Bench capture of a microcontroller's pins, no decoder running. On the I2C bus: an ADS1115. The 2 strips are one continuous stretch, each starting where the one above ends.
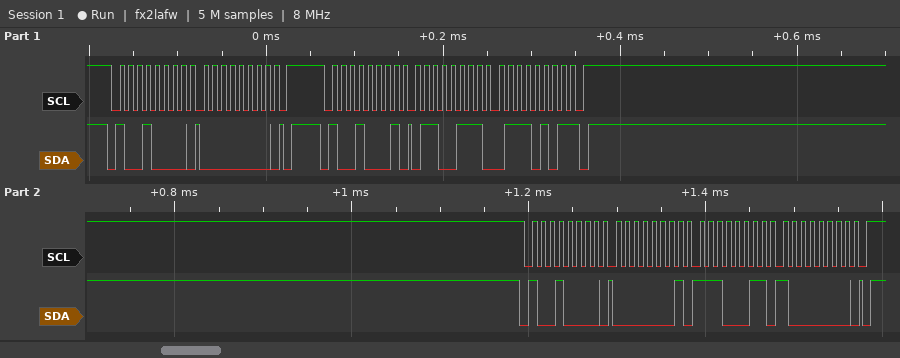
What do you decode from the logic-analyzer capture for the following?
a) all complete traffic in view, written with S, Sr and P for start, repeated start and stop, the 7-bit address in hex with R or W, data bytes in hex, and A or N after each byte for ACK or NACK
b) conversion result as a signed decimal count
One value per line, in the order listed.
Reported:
S 48W A 00 A P S 48R A 67 A 75 N P S 48W A 01 A E3 A 80 A P
26485
